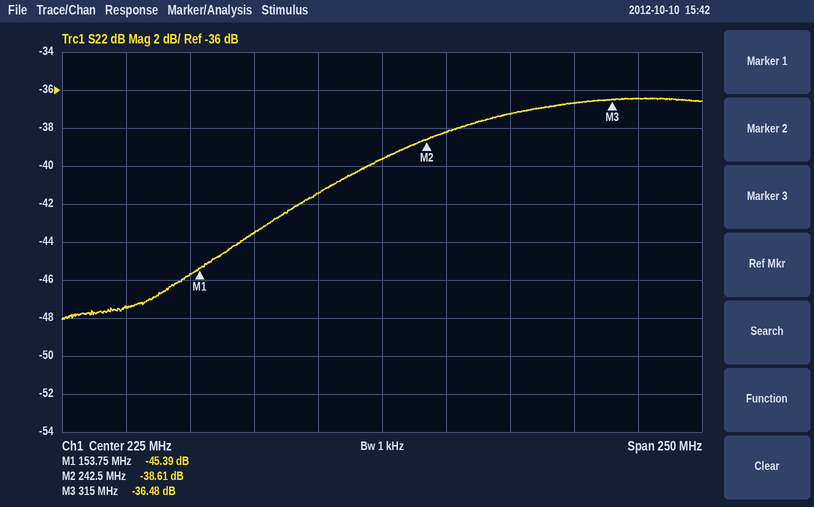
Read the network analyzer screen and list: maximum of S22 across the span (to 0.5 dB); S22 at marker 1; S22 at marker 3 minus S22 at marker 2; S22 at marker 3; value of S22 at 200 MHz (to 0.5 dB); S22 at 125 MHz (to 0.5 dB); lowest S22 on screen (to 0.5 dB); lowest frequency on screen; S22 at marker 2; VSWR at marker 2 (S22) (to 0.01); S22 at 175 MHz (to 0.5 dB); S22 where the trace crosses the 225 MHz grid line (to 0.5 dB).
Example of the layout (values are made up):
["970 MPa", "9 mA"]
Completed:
["-36.5 dB", "-45.39 dB", "2.13 dB", "-36.48 dB", "-41.5 dB", "-47.5 dB", "-48.0 dB", "100 MHz", "-38.61 dB", "1.02", "-43.5 dB", "-39.5 dB"]
